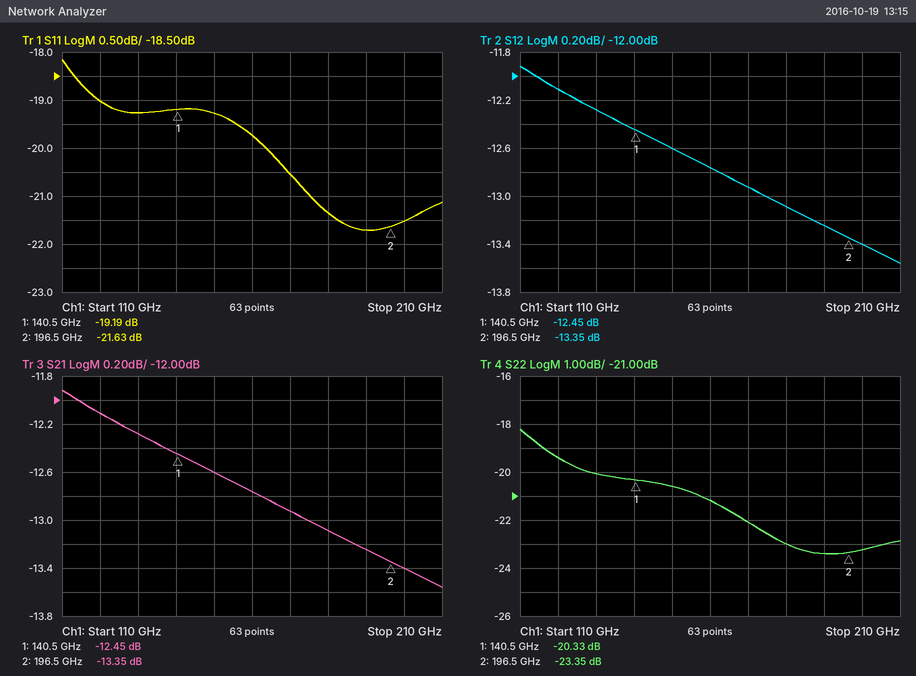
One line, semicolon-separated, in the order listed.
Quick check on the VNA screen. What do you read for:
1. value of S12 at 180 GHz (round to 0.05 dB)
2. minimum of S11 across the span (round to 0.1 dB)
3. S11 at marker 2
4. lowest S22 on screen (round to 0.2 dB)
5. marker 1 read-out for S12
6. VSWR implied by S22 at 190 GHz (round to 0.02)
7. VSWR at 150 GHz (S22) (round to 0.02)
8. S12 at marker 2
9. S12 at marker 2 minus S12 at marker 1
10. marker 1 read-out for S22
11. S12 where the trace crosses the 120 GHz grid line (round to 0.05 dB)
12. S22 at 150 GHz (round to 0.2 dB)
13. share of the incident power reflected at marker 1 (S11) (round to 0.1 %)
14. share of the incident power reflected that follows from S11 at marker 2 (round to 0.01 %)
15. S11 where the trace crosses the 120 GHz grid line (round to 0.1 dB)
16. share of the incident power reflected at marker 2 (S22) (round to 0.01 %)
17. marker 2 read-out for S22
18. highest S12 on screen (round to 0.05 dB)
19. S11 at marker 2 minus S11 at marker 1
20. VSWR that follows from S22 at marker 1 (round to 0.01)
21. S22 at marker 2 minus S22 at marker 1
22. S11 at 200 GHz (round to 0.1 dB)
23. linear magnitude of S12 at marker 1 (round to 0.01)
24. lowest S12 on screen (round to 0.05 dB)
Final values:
-13.10 dB; -21.7 dB; -21.63 dB; -23.4 dB; -12.45 dB; 1.14; 1.20; -13.35 dB; -0.90 dB; -20.33 dB; -12.10 dB; -20.6 dB; 1.2 %; 0.69 %; -19.0 dB; 0.46 %; -23.35 dB; -11.90 dB; -2.44 dB; 1.21; -3.02 dB; -21.5 dB; 0.24; -13.55 dB
